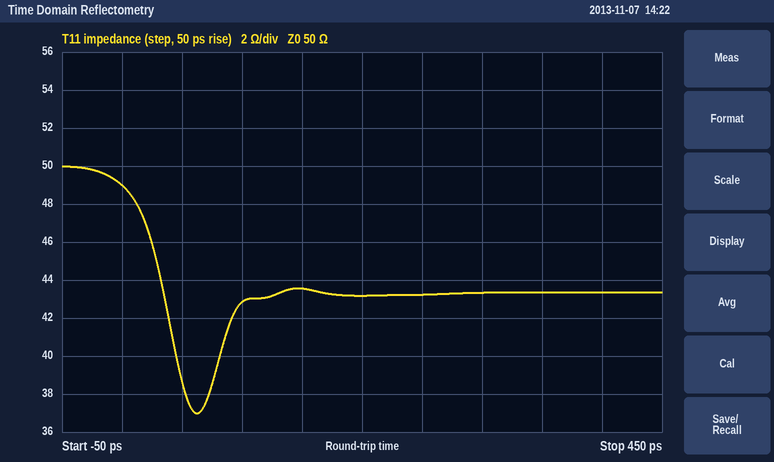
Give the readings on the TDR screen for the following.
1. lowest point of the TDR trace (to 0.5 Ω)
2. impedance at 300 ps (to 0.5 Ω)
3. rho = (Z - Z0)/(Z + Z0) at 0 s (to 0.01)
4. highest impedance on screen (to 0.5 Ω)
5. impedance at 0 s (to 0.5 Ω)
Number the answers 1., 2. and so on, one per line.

1. 37.0 Ω
2. 43.5 Ω
3. -0.01
4. 50.0 Ω
5. 49.0 Ω
